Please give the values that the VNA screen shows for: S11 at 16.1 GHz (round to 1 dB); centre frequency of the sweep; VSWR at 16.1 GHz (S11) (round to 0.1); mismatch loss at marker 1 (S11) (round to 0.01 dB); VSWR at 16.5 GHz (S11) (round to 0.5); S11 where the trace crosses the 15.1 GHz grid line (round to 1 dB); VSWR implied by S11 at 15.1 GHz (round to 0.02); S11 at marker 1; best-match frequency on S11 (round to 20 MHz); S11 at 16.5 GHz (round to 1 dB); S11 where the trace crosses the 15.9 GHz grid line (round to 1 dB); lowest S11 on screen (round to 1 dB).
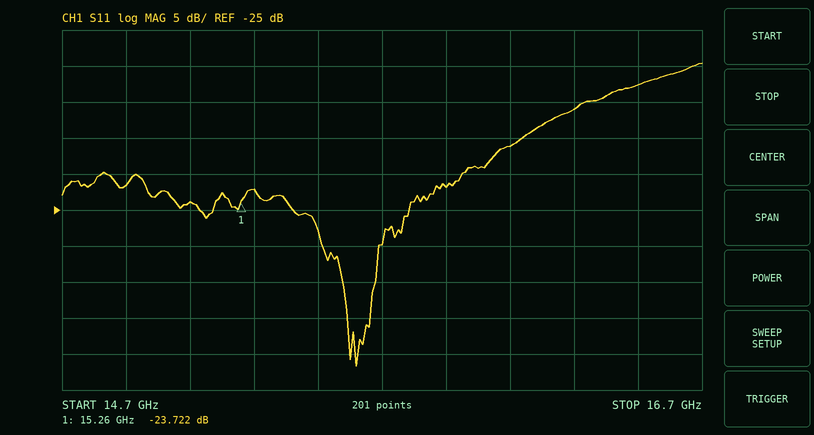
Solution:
-16 dB
15.7 GHz
1.4
0.02 dB
2.5
-24 dB
1.14
-23.722 dB
15.62 GHz
-8 dB
-22 dB
-47 dB
